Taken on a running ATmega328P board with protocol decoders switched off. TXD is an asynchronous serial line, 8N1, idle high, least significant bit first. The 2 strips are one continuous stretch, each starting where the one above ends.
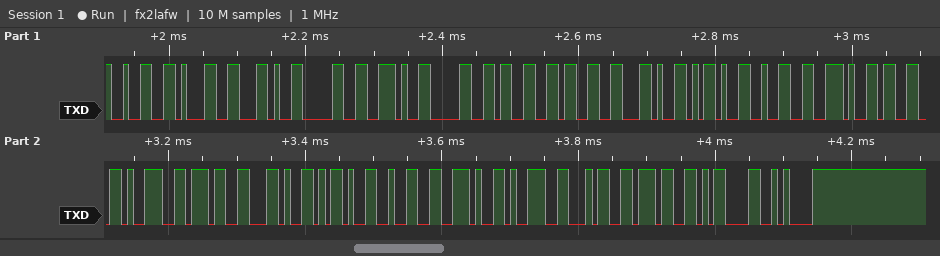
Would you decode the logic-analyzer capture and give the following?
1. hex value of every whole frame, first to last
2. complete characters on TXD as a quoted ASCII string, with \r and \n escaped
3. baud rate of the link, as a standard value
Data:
32 31 2C 30 2E 30 33 33 2C 2D 32 2E 33 39 37 2C 2D 32 2E 39 34 37 0D 0A
"21,0.033,-2.397,-2.947\r\n"
115200 baud
